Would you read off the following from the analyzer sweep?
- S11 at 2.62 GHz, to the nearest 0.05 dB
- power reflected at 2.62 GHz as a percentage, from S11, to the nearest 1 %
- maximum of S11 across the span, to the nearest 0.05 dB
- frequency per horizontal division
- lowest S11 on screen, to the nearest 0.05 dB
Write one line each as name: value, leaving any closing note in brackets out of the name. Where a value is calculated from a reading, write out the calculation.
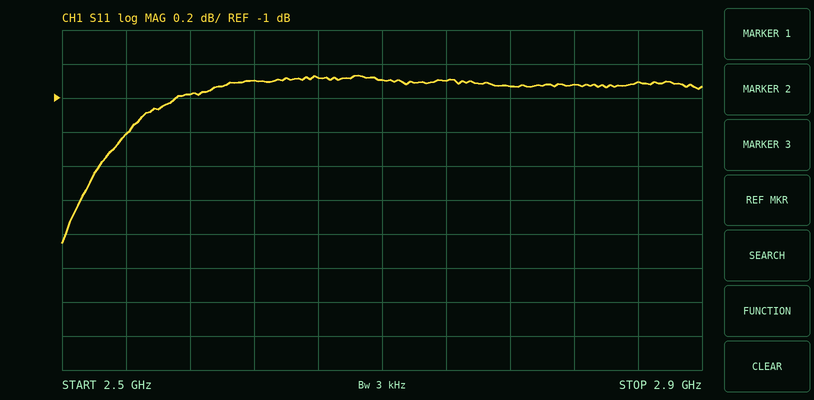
S11 at 2.62 GHz, to the nearest 0.05 dB: -0.90 dB
power reflected at 2.62 GHz as a percentage, from S11, to the nearest 1 %: 10^(-0.9/10) ≈ 81 %
maximum of S11 across the span, to the nearest 0.05 dB: -0.85 dB
frequency per horizontal division: 40 MHz
lowest S11 on screen, to the nearest 0.05 dB: -1.85 dB
